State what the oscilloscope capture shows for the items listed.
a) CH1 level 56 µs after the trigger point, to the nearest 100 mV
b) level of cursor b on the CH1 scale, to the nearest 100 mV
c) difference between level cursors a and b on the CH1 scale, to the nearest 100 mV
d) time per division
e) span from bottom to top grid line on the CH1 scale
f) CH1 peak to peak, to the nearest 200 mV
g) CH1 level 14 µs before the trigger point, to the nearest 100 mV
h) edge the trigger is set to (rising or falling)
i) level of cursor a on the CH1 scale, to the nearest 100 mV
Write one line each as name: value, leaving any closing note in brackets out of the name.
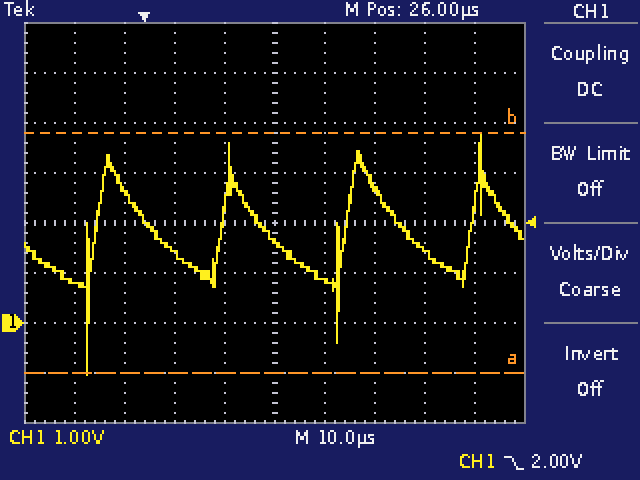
CH1 level 56 µs after the trigger point, to the nearest 100 mV: 1.5 V
level of cursor b on the CH1 scale, to the nearest 100 mV: 3.8 V
difference between level cursors a and b on the CH1 scale, to the nearest 100 mV: 4.8 V
time per division: 10 µs
span from bottom to top grid line on the CH1 scale: 8 V
CH1 peak to peak, to the nearest 200 mV: 4.8 V
CH1 level 14 µs before the trigger point, to the nearest 100 mV: 800 mV
edge the trigger is set to: falling
level of cursor a on the CH1 scale, to the nearest 100 mV: -1.0 V
